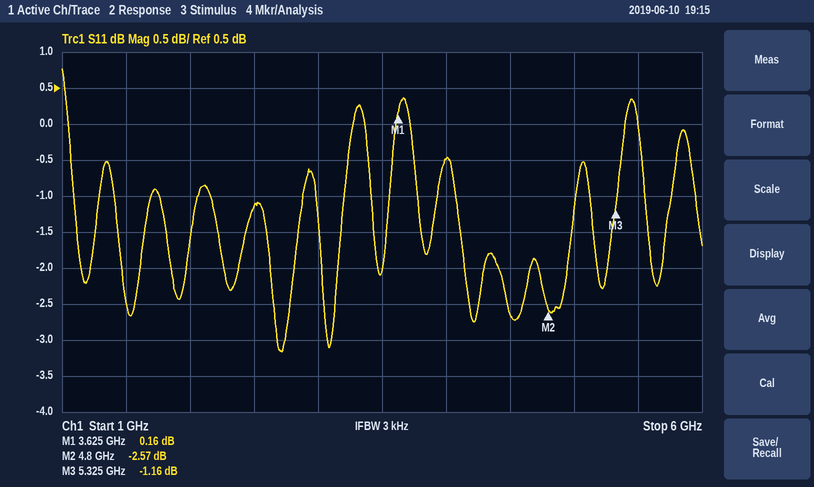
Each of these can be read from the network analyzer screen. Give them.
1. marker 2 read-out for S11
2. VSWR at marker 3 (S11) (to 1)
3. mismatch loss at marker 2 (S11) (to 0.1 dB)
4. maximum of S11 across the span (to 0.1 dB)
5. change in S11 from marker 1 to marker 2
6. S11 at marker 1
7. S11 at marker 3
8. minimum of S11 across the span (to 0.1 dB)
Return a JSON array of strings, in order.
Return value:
["-2.57 dB", "15", "3.5 dB", "0.8 dB", "-2.73 dB", "0.16 dB", "-1.16 dB", "-3.2 dB"]
